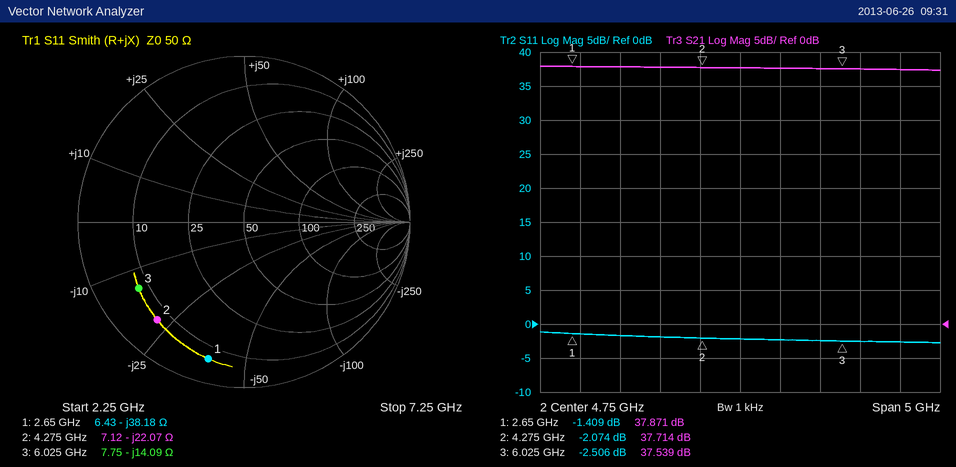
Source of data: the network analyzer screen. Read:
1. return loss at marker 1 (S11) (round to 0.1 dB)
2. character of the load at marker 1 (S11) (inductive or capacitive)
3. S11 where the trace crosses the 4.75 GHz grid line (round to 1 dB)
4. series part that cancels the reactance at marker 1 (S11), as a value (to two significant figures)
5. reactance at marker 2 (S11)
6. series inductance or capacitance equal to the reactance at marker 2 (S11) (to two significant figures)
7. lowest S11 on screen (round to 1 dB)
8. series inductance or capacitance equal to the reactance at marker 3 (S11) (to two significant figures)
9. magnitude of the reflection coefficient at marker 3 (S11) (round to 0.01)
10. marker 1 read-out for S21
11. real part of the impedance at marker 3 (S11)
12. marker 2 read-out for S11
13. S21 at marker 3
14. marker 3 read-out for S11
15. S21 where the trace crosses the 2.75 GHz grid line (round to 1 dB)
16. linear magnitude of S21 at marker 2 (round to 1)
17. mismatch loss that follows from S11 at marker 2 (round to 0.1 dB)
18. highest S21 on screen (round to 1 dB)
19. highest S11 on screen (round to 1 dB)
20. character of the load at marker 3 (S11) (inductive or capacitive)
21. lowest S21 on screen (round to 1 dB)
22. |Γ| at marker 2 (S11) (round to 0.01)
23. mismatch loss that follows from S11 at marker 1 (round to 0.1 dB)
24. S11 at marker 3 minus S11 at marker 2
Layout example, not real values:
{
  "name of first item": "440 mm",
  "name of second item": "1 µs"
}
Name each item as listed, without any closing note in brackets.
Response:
{
  "return loss at marker 1 (S11)": "1.4 dB",
  "character of the load at marker 1 (S11)": "capacitive",
  "S11 where the trace crosses the 4.75 GHz grid line": "-2 dB",
  "series part that cancels the reactance at marker 1 (S11), as a value": "2.3 nH",
  "reactance at marker 2": "-22.07 Ω",
  "series inductance or capacitance equal to the reactance at marker 2 (S11)": "1.7 pF",
  "lowest S11 on screen": "-3 dB",
  "series inductance or capacitance equal to the reactance at marker 3 (S11)": "1.9 pF",
  "magnitude of the reflection coefficient at marker 3 (S11)": "0.75",
  "marker 1 read-out for S21": "37.871 dB",
  "real part of the impedance at marker 3": "7.75 Ω",
  "marker 2 read-out for S11": "-2.074 dB",
  "S21 at marker 3": "37.539 dB",
  "marker 3 read-out for S11": "-2.506 dB",
  "S21 where the trace crosses the 2.75 GHz grid line": "38 dB",
  "linear magnitude of S21 at marker 2": "77",
  "mismatch loss that follows from S11 at marker 2": "4.2 dB",
  "highest S21 on screen": "38 dB",
  "highest S11 on screen": "-1 dB",
  "character of the load at marker 3 (S11)": "capacitive",
  "lowest S21 on screen": "37 dB",
  "|Γ| at marker 2 (S11)": "0.79",
  "mismatch loss that follows from S11 at marker 1": "5.6 dB",
  "S11 at marker 3 minus S11 at marker 2": "-0.432 dB"
}
